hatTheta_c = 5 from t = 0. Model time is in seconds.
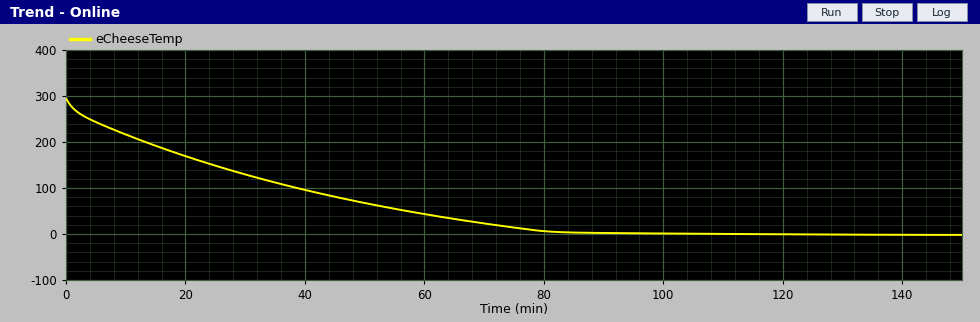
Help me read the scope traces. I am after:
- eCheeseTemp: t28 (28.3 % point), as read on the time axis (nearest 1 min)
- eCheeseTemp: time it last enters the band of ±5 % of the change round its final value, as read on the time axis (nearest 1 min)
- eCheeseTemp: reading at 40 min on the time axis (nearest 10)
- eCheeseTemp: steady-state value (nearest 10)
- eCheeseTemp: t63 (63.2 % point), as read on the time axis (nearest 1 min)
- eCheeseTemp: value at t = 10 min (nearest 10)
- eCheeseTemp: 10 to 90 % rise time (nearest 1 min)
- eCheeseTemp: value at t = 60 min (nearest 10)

11 min
76 min
100
0
36 min
220
66 min
40
